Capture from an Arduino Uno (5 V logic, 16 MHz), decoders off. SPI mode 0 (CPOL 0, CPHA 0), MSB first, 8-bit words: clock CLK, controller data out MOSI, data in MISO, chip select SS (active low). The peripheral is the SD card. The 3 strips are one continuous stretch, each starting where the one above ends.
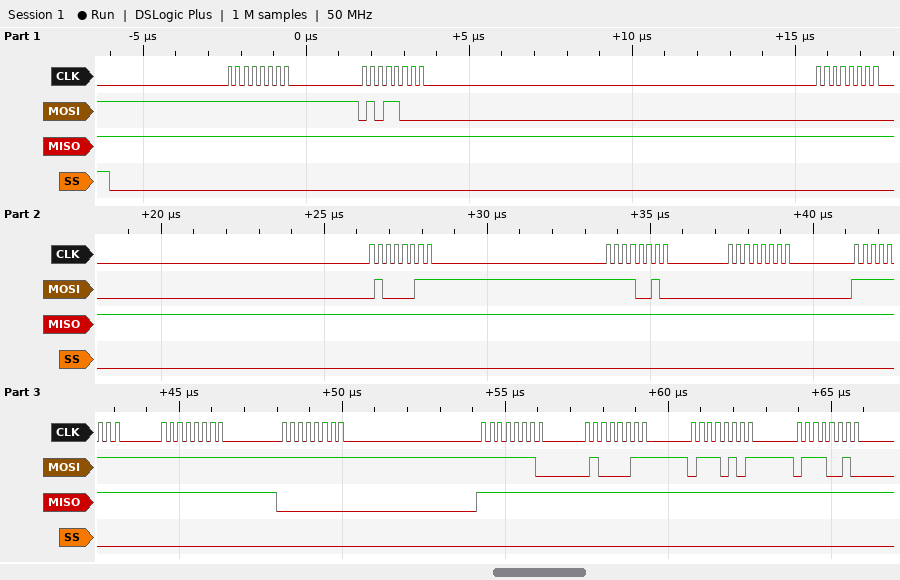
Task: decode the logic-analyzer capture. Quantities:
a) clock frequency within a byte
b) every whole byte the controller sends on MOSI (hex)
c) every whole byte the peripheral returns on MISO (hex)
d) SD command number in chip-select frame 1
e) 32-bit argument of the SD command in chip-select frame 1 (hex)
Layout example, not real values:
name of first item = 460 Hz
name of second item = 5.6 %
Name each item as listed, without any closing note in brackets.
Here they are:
clock frequency within a byte = 4 MHz
every whole byte the controller sends on MOSI = FF 58 00 43 F2 00 FF FF FF FE 43 75 72
every whole byte the peripheral returns on MISO = FF FF FF FF FF FF FF FF 00 FF FF FF FF
SD command number in chip-select frame 1 = CMD24
32-bit argument of the SD command in chip-select frame 1 = 0x0043F200
